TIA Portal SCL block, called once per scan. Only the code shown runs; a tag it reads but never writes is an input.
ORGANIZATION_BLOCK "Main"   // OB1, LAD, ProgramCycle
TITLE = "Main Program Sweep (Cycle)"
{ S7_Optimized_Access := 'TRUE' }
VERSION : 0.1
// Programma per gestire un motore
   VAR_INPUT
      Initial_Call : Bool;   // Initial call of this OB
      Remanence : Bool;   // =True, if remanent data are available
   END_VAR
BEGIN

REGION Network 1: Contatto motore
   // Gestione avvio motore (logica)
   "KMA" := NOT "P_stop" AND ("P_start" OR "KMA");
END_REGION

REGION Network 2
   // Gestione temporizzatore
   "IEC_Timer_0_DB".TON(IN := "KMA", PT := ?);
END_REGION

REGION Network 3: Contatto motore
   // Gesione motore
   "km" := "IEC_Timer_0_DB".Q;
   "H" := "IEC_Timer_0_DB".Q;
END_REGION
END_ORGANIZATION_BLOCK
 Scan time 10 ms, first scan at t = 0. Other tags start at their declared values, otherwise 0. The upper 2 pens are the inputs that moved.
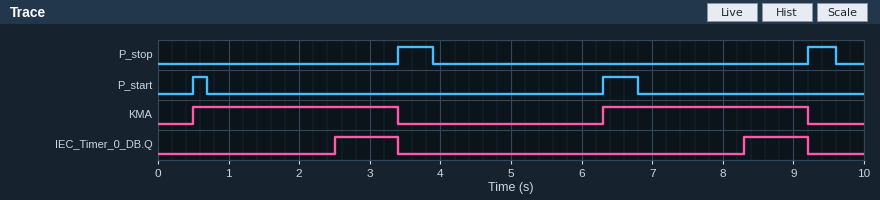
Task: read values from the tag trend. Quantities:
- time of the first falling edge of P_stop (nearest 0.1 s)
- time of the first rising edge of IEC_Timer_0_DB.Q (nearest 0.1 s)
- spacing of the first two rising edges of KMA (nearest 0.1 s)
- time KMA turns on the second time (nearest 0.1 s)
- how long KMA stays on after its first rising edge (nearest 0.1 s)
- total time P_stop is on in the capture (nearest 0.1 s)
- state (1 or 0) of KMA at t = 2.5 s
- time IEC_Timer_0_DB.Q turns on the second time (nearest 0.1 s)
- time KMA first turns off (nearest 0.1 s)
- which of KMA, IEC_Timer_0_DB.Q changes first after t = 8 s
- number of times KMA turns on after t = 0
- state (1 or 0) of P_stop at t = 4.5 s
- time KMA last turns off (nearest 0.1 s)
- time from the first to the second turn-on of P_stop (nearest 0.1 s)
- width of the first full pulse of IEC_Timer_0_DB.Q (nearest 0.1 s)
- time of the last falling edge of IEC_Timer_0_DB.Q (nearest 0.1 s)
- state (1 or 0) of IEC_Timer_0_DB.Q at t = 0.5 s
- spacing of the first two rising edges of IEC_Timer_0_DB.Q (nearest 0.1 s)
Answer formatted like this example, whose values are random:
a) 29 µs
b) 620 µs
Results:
a) 3.9 s
b) 2.5 s
c) 5.8 s
d) 6.3 s
e) 2.9 s
f) 0.9 s
g) 1
h) 8.3 s
i) 3.4 s
j) IEC_Timer_0_DB.Q
k) 2
l) 0
m) 9.2 s
n) 5.8 s
o) 0.9 s
p) 9.2 s
q) 0
r) 5.8 s
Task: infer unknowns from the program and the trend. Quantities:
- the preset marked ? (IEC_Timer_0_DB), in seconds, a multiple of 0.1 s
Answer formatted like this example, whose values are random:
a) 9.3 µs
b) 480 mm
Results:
a) 2.0 s
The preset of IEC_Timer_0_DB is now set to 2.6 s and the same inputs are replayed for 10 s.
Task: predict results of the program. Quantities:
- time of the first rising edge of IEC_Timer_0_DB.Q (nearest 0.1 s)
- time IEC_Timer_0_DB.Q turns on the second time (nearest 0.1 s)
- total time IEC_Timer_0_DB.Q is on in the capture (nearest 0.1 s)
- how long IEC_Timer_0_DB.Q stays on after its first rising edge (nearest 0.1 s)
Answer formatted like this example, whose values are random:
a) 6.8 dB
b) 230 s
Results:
a) 3.1 s
b) 8.9 s
c) 0.6 s
d) 0.3 s
